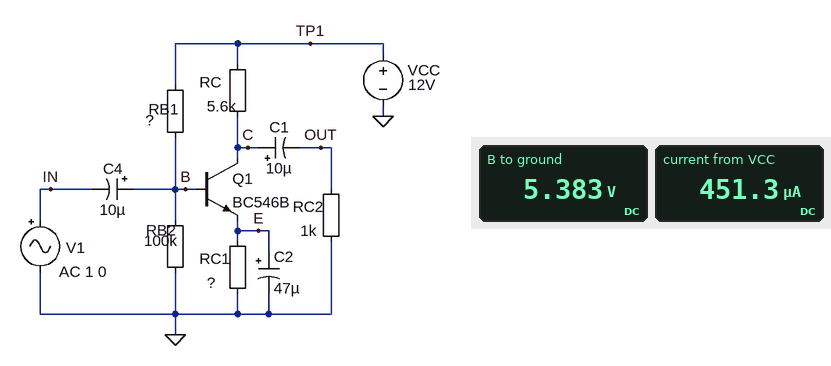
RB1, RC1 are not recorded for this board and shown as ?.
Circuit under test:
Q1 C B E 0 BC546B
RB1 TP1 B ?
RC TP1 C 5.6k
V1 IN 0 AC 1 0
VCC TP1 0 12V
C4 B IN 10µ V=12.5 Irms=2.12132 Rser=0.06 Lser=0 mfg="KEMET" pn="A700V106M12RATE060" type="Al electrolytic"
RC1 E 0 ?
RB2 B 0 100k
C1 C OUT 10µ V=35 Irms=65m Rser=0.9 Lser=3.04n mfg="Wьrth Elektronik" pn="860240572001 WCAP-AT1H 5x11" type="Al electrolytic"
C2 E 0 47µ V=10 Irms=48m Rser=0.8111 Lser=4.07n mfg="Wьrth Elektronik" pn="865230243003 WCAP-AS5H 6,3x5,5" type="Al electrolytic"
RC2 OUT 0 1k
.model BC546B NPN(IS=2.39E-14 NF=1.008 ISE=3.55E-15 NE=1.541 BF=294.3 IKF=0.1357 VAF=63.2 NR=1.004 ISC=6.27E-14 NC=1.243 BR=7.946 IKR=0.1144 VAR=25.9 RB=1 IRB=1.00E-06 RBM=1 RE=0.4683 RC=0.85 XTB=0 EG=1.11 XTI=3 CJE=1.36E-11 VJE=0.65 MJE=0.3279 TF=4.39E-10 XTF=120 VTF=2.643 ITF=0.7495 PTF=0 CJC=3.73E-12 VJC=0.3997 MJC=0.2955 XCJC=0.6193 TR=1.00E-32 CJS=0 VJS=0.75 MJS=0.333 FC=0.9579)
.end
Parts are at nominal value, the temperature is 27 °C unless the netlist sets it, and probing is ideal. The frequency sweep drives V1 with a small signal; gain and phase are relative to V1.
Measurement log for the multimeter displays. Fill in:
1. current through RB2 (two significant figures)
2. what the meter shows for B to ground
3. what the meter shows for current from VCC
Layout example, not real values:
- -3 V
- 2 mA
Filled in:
- 54 µA
- 5.383 V
- 451.3 µA
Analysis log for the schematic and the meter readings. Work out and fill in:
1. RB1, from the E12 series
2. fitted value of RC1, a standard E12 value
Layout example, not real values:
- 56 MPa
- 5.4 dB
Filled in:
- 120 kΩ
- 12 kΩ
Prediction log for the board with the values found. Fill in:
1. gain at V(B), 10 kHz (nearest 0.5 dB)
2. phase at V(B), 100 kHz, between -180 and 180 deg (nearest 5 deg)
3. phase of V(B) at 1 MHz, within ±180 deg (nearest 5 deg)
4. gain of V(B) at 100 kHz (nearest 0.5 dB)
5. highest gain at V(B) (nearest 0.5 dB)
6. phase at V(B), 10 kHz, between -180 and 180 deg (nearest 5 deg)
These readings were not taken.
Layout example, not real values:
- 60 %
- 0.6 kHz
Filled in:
- 0 dB
- 0 deg
- 0 deg
- 0 dB
- 0 dB
- 0 deg
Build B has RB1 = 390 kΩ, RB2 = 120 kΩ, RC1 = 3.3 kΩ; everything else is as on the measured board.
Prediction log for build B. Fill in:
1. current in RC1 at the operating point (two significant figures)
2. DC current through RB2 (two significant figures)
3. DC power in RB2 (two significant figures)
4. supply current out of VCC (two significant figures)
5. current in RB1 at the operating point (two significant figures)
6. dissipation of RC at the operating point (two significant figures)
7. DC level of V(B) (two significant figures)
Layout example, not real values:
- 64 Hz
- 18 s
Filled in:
- 610 µA
- 22 µA
- 58 µW
- 630 µA
- 24 µA
- 2.1 mW
- 2.6 V
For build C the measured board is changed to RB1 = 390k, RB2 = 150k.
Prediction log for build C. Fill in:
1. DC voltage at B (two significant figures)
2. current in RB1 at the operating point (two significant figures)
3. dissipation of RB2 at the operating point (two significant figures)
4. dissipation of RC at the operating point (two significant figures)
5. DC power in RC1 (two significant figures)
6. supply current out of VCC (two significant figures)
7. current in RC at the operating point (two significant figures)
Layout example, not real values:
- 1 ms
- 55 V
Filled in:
- 3.3 V
- 22 µA
- 71 µW
- 270 µW
- 590 µW
- 240 µA
- 220 µA
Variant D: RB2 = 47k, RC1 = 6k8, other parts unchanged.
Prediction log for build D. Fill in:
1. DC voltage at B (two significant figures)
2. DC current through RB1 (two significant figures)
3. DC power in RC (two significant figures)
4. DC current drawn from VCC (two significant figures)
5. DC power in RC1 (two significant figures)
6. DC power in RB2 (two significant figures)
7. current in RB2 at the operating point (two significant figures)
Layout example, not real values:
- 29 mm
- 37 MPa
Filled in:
- 3.3 V
- 72 µA
- 890 µW
- 470 µA
- 1.1 mW
- 240 µW
- 71 µA
